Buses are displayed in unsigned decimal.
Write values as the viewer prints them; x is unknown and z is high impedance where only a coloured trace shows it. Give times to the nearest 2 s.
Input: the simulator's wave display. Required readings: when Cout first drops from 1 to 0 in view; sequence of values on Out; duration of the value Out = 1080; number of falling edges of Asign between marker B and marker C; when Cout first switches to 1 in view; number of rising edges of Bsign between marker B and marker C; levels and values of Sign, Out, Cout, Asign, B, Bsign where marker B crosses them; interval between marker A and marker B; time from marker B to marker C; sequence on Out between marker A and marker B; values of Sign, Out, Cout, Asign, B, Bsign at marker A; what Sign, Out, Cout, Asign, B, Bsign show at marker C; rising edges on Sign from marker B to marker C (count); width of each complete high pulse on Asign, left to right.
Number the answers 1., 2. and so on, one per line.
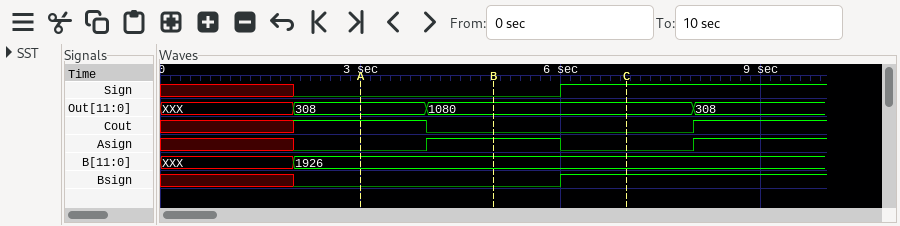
1. 4 s
2. XXX, 308, 1080, 308
3. 4 s
4. 1
5. 2 s
6. 1
7. Sign=0, Out=1080, Cout=0, Asign=1, B=1926, Bsign=0
8. 2 s
9. 2 s
10. 308, 1080
11. Sign=0, Out=308, Cout=1, Asign=0, B=1926, Bsign=0
12. Sign=1, Out=1080, Cout=0, Asign=0, B=1926, Bsign=1
13. 1
14. 2 s
